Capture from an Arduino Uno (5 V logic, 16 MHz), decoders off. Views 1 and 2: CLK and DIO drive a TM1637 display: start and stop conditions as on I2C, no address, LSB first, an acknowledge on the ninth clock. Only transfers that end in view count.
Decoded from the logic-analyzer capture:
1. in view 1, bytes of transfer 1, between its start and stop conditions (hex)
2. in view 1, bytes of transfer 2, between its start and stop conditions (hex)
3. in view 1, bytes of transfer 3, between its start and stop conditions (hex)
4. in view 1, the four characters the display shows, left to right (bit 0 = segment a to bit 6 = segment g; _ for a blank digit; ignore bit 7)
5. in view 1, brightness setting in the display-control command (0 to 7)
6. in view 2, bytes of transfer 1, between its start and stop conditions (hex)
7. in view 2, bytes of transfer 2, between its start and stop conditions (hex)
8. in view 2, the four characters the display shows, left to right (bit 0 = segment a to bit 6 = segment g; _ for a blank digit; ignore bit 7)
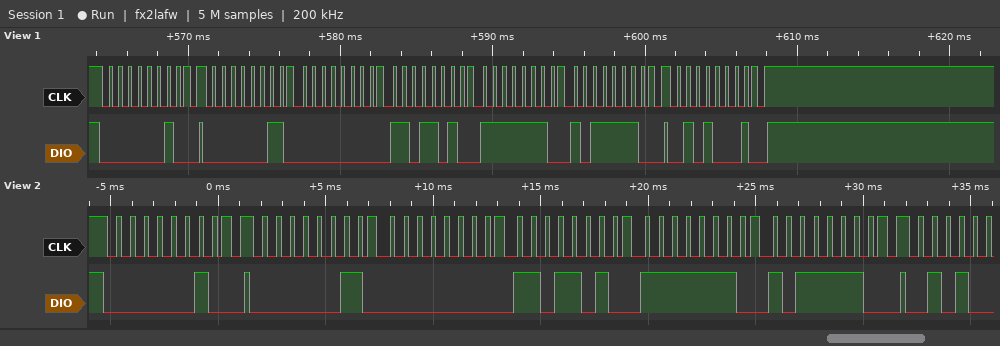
40
C0 00 5B 7F 7D
8A
_286
2
40
C0 00 5B 7F 7D
_286
